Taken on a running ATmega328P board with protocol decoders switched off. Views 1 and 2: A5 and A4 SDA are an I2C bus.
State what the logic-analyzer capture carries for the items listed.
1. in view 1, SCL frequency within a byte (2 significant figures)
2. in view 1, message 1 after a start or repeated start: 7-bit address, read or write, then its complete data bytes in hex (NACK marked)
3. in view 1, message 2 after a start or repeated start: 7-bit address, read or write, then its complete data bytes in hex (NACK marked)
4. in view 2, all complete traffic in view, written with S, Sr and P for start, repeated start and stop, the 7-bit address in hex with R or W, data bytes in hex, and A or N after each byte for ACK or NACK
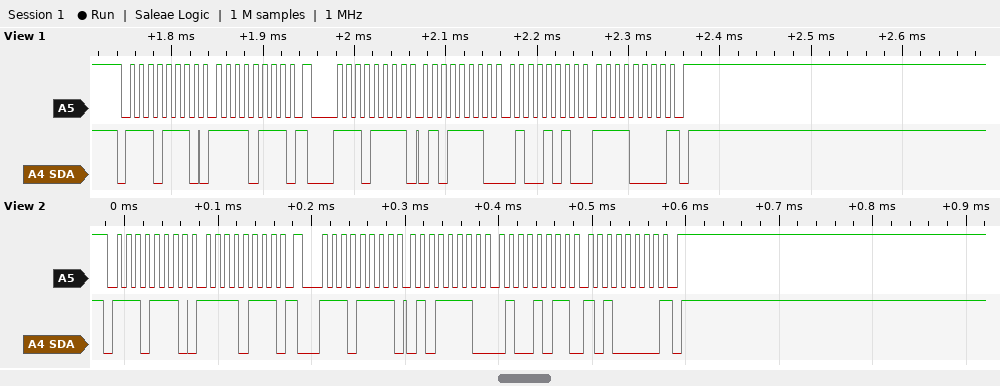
100 kHz
0x77 write: F7
0x77 read: 5E 4A F0 NACK
S 77W A F7 A Sr 77R A 5E A 4B A A0 N P
